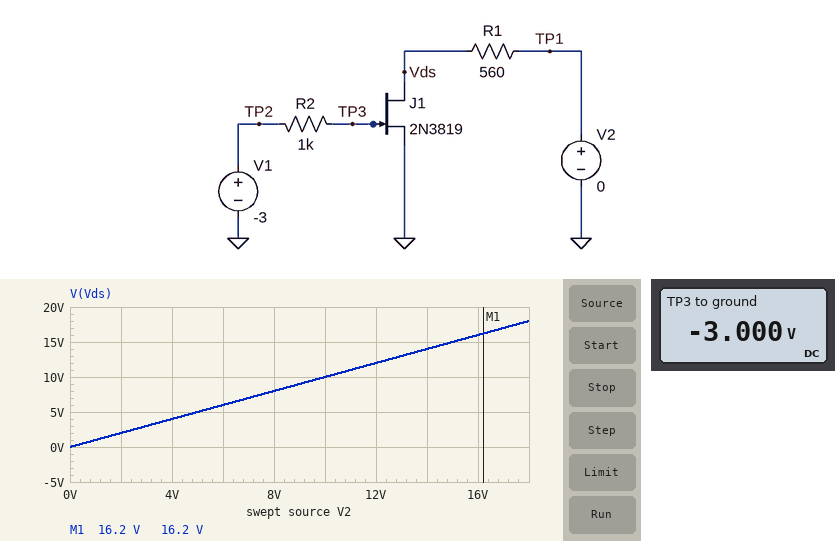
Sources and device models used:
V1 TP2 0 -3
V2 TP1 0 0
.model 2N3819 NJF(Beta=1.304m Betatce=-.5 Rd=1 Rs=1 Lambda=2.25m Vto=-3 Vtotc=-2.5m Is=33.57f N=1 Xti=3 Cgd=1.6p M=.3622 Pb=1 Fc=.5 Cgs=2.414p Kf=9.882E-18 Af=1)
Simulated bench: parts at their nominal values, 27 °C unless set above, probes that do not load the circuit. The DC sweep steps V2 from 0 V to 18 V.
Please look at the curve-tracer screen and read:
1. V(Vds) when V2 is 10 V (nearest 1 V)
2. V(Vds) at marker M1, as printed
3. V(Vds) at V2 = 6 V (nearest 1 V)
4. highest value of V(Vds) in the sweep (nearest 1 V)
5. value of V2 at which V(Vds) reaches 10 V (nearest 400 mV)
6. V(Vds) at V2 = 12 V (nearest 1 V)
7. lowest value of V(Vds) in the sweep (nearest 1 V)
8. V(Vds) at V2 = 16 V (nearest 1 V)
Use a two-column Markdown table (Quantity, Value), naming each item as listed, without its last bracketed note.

| Quantity | Value |
|---|---|
| V(Vds) when V2 is 10 V | 10 V |
| V(Vds) at marker M1, as printed | 16.2 V |
| V(Vds) at V2 = 6 V | 6 V |
| highest value of V(Vds) in the sweep | 18 V |
| value of V2 at which V(Vds) reaches 10 V | 10.0 V |
| V(Vds) at V2 = 12 V | 12 V |
| lowest value of V(Vds) in the sweep | 0 V |
| V(Vds) at V2 = 16 V | 16 V |
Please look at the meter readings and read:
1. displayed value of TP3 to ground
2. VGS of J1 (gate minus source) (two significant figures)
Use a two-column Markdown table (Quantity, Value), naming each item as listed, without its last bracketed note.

| Quantity | Value |
|---|---|
| displayed value of TP3 to ground | -3.000 V |
| VGS of J1 (gate minus source) | -3.0 V |
